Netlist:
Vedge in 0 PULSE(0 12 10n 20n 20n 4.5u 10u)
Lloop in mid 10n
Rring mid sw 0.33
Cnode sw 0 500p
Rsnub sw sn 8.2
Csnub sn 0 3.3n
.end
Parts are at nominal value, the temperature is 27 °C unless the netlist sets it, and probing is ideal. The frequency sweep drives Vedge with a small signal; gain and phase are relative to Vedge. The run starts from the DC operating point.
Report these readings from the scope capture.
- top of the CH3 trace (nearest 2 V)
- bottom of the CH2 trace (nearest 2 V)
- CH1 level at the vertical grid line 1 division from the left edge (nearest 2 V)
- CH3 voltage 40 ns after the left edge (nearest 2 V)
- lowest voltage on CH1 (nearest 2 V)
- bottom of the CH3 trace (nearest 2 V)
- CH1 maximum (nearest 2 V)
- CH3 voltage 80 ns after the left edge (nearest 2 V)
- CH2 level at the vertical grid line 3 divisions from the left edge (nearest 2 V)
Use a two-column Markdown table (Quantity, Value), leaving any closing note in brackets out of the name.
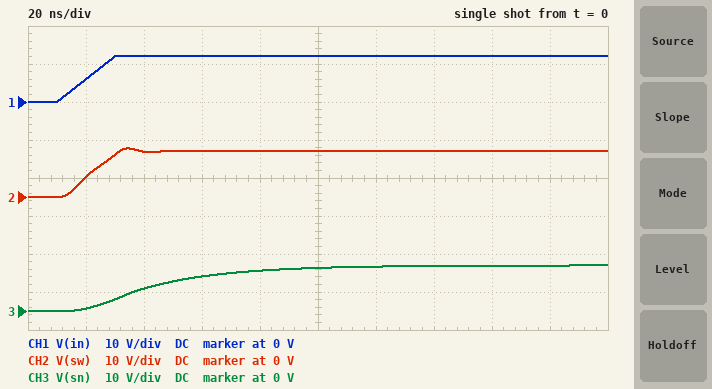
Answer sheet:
| Quantity | Value |
|---|---|
| top of the CH3 trace | 12 V |
| bottom of the CH2 trace | 0 V |
| CH1 level at the vertical grid line 1 division from the left edge | 6 V |
| CH3 voltage 40 ns after the left edge | 6 V |
| lowest voltage on CH1 | 0 V |
| bottom of the CH3 trace | 0 V |
| CH1 maximum | 12 V |
| CH3 voltage 80 ns after the left edge | 10 V |
| CH2 level at the vertical grid line 3 divisions from the left edge | 12 V |
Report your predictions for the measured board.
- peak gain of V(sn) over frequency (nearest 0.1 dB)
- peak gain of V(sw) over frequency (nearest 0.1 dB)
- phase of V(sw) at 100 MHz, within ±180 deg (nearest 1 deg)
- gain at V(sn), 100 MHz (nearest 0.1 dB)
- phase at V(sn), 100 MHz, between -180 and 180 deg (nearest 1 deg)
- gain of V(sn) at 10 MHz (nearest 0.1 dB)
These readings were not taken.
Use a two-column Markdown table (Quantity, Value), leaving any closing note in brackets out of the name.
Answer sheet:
| Quantity | Value |
|---|---|
| peak gain of V(sn) over frequency | 0 dB |
| peak gain of V(sw) over frequency | 4.6 dB |
| phase of V(sw) at 100 MHz, within ±180 deg | -138 deg |
| gain at V(sn), 100 MHz | -27.0 dB |
| phase at V(sn), 100 MHz, between -180 and 180 deg | 135 deg |
| gain of V(sn) at 10 MHz | -5.7 dB |
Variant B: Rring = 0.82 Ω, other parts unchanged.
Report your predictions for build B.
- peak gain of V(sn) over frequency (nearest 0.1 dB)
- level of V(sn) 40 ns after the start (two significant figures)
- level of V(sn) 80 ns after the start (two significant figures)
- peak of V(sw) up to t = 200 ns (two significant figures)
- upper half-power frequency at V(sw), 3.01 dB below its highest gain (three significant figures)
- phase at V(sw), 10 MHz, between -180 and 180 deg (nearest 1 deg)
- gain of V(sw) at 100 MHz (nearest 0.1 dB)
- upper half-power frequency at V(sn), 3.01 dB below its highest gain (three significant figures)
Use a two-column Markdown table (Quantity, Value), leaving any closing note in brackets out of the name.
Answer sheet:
| Quantity | Value |
|---|---|
| peak gain of V(sn) over frequency | 0 dB |
| level of V(sn) 40 ns after the start | 5.6 V |
| level of V(sn) 80 ns after the start | 10 V |
| peak of V(sw) up to t = 200 ns | 12 V |
| upper half-power frequency at V(sw), 3.01 dB below its highest gain | 87.0 MHz |
| phase at V(sw), 10 MHz, between -180 and 180 deg | -7 deg |
| gain of V(sw) at 100 MHz | -2.8 dB |
| upper half-power frequency at V(sn), 3.01 dB below its highest gain | 5.61 MHz |
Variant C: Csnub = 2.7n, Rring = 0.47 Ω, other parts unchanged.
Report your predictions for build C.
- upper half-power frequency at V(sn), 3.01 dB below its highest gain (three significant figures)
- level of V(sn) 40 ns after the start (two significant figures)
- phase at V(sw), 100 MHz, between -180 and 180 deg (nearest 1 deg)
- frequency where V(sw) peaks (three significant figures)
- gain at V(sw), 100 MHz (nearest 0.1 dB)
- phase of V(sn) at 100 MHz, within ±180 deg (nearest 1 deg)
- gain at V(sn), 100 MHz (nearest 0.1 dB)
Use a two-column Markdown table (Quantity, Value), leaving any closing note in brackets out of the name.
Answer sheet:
| Quantity | Value |
|---|---|
| upper half-power frequency at V(sn), 3.01 dB below its highest gain | 7.29 MHz |
| level of V(sn) 40 ns after the start | 6.7 V |
| phase at V(sw), 100 MHz, between -180 and 180 deg | -137 deg |
| frequency where V(sw) peaks | 63.3 MHz |
| gain at V(sw), 100 MHz | -2.5 dB |
| phase of V(sn) at 100 MHz, within ±180 deg | 137 deg |
| gain at V(sn), 100 MHz | -25.4 dB |
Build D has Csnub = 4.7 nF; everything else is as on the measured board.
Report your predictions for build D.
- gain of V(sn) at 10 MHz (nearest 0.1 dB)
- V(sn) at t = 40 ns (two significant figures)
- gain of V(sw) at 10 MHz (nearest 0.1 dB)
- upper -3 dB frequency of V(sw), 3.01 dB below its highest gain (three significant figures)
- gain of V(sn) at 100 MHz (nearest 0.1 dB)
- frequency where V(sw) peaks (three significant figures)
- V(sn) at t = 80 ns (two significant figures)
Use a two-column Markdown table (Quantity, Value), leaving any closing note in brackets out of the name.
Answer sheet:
| Quantity | Value |
|---|---|
| gain of V(sn) at 10 MHz | -8.3 dB |
| V(sn) at t = 40 ns | 4.5 V |
| gain of V(sw) at 10 MHz | 0.1 dB |
| upper -3 dB frequency of V(sw), 3.01 dB below its highest gain | 84.5 MHz |
| gain of V(sn) at 100 MHz | -30.0 dB |
| frequency where V(sw) peaks | 64.3 MHz |
| V(sn) at t = 80 ns | 9.3 V |
